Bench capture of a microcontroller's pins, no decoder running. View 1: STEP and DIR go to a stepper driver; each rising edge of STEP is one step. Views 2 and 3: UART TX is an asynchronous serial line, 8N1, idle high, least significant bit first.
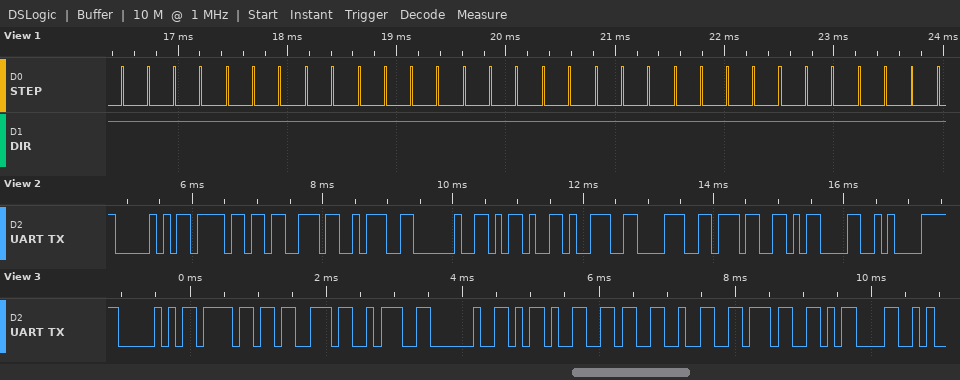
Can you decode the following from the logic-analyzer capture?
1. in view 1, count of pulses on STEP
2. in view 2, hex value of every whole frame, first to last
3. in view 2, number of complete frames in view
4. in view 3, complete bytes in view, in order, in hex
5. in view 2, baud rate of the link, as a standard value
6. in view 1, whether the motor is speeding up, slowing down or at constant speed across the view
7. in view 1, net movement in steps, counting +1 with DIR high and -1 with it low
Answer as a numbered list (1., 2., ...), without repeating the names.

1. 32
2. 50 6F 73 3A 20 2D 39 38 37 0D 0A
3. 11
4. 50 6F 73 3A 20 2D 36 32 37 0D
5. 9600 baud
6. constant speed
7. +32
